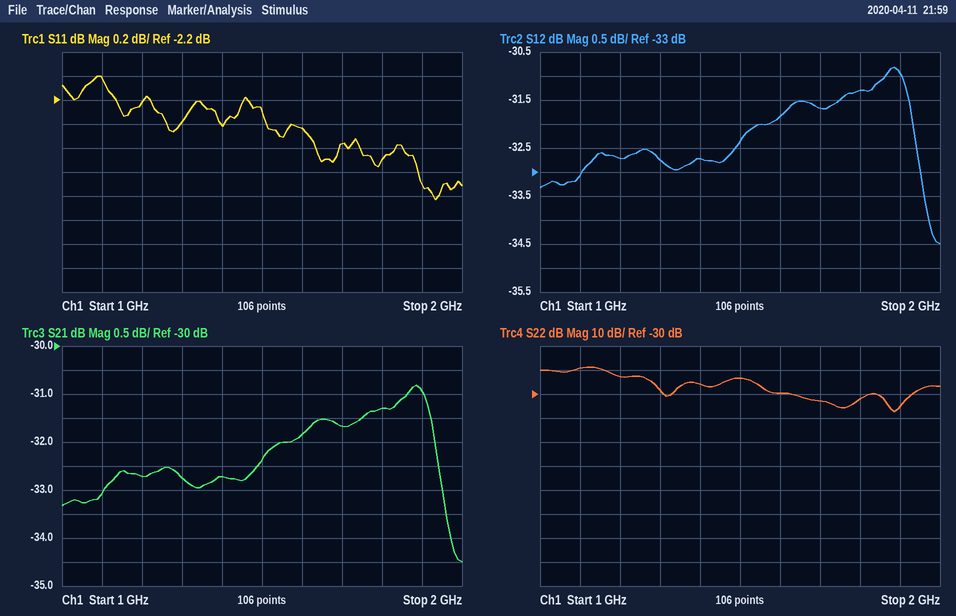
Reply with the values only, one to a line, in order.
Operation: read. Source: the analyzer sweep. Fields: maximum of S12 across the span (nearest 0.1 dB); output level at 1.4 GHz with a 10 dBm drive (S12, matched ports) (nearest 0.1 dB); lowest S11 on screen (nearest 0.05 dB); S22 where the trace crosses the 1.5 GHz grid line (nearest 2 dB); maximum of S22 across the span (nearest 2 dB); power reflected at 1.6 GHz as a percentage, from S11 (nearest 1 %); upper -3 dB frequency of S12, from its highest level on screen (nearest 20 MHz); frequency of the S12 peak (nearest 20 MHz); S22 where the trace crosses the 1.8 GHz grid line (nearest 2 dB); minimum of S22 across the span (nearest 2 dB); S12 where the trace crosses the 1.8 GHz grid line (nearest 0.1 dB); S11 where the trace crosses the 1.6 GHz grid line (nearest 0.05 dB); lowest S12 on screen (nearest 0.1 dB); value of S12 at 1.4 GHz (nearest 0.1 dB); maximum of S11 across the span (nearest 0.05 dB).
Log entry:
-30.8 dB
-22.7 dBm
-3.05 dB
-24 dB
-18 dB
57 %
1.96 GHz
1.88 GHz
-32 dB
-38 dB
-31.3 dB
-2.45 dB
-34.5 dB
-32.7 dB
-2.00 dB
